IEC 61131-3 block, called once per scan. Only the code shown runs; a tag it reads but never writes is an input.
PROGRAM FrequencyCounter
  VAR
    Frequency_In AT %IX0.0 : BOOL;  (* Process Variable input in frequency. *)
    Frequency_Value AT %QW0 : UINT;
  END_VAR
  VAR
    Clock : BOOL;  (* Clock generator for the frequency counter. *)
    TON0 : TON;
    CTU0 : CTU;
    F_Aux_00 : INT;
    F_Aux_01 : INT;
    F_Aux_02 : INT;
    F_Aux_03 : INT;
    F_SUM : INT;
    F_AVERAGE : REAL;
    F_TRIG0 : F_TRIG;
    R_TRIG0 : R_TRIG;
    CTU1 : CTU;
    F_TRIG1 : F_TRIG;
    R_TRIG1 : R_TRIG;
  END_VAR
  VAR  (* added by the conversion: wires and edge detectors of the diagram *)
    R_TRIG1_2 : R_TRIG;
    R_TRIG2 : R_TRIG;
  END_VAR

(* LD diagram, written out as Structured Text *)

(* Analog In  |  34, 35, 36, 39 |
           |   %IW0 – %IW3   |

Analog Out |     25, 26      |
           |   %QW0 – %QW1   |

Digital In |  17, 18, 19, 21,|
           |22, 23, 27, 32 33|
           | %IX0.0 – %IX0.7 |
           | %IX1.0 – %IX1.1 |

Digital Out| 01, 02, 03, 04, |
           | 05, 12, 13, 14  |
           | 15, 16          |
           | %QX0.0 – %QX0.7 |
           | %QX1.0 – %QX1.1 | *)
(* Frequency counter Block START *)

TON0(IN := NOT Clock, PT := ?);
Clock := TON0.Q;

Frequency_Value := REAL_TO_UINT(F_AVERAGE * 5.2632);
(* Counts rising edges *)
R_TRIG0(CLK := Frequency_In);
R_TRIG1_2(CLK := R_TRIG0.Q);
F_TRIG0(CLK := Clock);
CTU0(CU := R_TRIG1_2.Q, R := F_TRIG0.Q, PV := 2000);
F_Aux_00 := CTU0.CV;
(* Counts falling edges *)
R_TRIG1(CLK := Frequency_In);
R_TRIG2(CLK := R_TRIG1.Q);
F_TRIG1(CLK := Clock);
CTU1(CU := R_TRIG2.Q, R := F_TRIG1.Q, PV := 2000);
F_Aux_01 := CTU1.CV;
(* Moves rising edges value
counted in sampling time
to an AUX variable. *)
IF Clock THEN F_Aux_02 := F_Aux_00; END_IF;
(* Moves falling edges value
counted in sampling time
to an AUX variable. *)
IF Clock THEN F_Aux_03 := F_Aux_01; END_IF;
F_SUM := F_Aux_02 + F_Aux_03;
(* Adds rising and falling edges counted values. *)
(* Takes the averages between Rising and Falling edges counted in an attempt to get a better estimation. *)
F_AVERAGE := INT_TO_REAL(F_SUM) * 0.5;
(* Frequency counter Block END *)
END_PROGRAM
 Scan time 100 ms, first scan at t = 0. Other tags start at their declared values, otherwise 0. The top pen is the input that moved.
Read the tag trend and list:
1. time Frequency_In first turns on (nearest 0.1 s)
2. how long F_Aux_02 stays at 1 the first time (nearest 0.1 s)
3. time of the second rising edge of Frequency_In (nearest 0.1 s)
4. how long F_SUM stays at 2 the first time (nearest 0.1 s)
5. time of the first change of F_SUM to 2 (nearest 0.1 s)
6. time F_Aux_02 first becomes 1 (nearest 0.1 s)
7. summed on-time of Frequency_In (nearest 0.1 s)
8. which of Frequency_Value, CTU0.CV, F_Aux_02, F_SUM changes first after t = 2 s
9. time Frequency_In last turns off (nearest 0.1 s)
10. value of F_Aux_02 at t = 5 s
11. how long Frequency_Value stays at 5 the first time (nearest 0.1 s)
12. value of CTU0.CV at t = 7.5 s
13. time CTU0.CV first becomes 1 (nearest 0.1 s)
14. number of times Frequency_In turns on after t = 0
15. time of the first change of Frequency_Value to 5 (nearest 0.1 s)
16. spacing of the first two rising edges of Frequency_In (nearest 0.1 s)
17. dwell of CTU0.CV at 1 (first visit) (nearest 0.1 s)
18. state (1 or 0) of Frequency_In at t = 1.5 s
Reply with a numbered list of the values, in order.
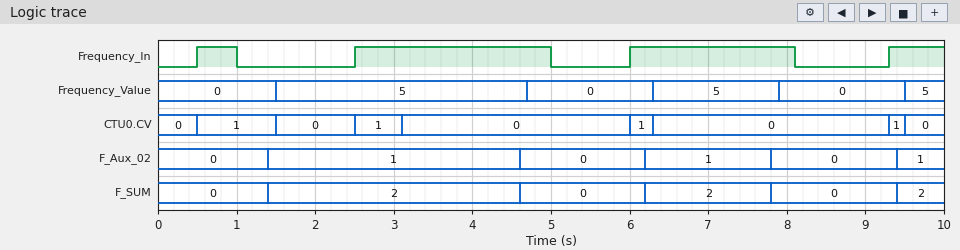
1. 0.5 s
2. 3.2 s
3. 2.5 s
4. 3.2 s
5. 1.4 s
6. 1.4 s
7. 5.8 s
8. CTU0.CV
9. 8.1 s
10. 0
11. 3.2 s
12. 0
13. 0.5 s
14. 4
15. 1.5 s
16. 2.0 s
17. 1.0 s
18. 0
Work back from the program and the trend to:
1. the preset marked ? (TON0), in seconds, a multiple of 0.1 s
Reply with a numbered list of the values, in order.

1. 1.4 s
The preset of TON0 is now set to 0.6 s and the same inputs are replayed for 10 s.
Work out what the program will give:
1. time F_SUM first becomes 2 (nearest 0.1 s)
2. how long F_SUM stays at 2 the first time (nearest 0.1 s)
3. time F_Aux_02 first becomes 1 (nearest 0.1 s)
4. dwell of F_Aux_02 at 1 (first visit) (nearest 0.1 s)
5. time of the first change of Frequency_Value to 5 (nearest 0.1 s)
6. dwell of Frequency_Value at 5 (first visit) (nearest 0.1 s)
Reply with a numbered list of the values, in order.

1. 0.6 s
2. 0.8 s
3. 0.6 s
4. 0.8 s
5. 0.7 s
6. 0.8 s
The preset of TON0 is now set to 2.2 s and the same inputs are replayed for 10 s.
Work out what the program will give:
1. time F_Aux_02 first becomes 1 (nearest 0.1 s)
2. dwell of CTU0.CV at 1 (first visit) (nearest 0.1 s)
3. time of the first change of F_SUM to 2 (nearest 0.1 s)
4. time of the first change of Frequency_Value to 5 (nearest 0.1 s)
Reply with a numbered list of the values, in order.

1. 2.2 s
2. 1.8 s
3. 2.2 s
4. 2.3 s
